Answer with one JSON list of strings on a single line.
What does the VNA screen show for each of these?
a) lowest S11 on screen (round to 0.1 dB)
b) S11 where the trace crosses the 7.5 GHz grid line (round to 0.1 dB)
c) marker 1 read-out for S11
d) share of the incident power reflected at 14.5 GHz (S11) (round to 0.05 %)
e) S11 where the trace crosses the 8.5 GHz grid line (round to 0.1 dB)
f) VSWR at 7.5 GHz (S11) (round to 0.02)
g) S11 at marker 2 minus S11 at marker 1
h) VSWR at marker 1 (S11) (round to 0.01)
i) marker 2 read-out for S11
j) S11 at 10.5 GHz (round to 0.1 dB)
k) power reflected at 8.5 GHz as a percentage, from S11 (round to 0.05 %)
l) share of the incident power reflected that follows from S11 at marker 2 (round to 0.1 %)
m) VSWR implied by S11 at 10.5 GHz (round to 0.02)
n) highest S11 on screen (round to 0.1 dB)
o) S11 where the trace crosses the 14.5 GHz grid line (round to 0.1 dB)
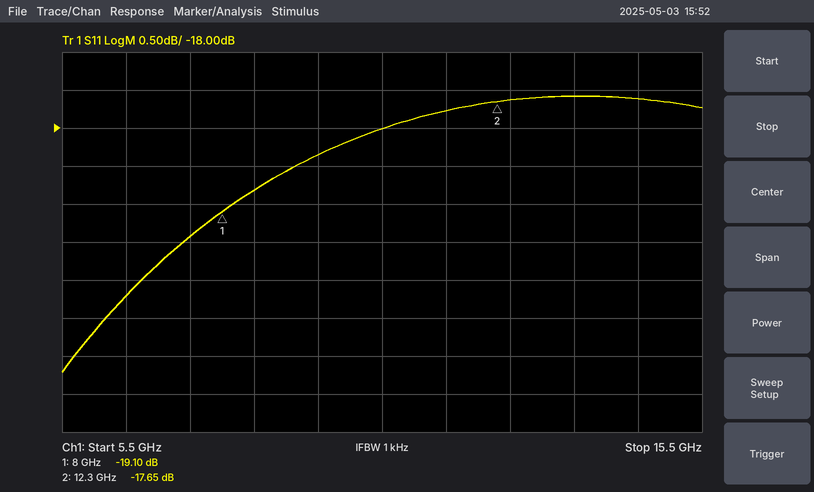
["-21.2 dB", "-19.4 dB", "-19.10 dB", "1.75 %", "-18.8 dB", "1.24", "1.45 dB", "1.25", "-17.65 dB", "-18.0 dB", "1.30 %", "1.7 %", "1.28", "-17.6 dB", "-17.6 dB"]
